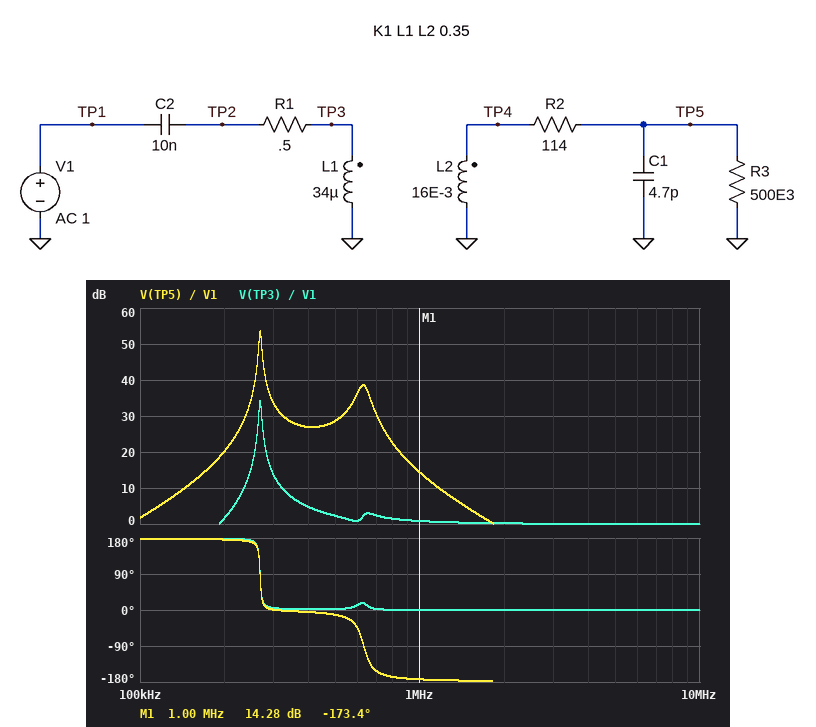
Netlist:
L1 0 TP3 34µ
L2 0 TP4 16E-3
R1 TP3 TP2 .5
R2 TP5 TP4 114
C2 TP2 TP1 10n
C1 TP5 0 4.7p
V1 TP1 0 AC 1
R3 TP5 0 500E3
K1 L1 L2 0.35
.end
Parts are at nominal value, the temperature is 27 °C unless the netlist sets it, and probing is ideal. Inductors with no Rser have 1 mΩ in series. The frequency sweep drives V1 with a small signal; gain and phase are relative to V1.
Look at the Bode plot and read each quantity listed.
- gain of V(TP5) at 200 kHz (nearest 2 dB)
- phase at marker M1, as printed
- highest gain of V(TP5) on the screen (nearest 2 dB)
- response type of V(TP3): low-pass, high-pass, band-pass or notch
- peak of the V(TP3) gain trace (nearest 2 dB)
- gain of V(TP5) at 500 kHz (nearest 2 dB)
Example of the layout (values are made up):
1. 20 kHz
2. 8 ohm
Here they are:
1. 20 dB
2. -173.4 deg
3. 54 dB
4. band-pass
5. 34 dB
6. 28 dB
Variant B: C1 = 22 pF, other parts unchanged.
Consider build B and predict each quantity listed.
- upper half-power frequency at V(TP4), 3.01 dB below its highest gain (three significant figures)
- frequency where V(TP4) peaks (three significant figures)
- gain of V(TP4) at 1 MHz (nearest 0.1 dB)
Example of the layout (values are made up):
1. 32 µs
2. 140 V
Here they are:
1. 340 kHz
2. 335 kHz
3. -2.6 dB
